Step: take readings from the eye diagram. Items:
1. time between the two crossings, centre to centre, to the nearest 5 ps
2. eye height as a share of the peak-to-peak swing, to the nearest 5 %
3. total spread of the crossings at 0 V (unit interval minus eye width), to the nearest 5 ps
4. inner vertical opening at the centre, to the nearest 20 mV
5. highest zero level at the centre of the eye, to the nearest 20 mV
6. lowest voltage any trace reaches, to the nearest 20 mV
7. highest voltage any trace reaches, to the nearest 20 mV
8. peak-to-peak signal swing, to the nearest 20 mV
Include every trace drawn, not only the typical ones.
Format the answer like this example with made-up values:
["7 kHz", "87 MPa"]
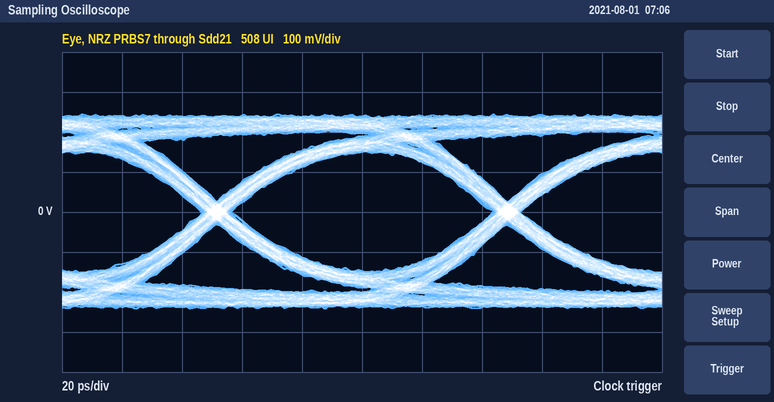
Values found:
["95 ps", "60 %", "10 ps", "300 mV", "-140 mV", "-240 mV", "240 mV", "480 mV"]
